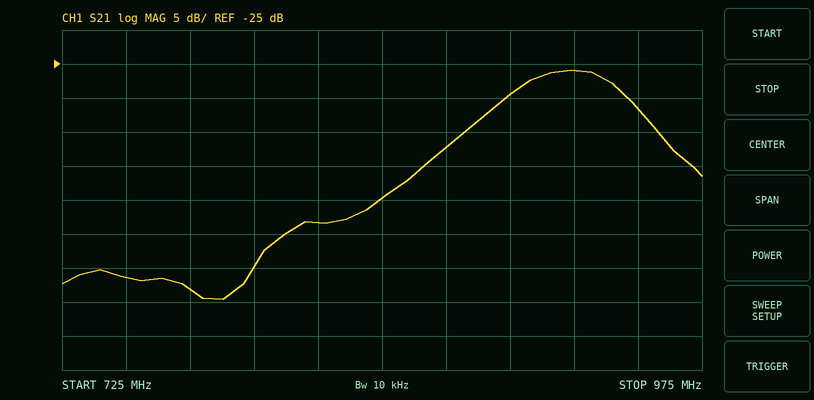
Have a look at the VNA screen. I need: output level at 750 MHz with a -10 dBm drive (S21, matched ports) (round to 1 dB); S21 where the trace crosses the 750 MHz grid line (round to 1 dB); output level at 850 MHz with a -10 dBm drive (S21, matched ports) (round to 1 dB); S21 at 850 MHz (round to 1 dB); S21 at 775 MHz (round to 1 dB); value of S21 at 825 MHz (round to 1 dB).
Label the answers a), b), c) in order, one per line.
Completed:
a) -66 dBm
b) -56 dB
c) -55 dBm
d) -45 dB
e) -58 dB
f) -48 dB
